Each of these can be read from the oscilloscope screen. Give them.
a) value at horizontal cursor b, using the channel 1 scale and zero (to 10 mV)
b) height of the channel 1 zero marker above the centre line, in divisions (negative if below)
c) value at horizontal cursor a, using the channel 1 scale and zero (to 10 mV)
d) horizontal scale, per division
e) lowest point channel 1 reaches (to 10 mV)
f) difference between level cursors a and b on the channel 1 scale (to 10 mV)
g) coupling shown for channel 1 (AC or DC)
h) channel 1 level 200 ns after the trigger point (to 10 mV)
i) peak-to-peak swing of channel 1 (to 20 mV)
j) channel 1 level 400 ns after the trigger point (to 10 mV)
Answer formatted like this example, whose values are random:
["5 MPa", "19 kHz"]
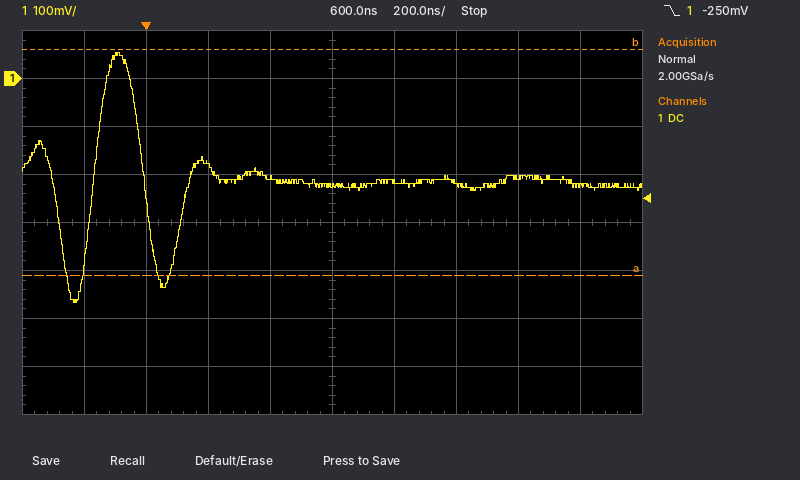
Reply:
["60 mV", "+3.0 div", "-410 mV", "200 ns", "-470 mV", "470 mV", "DC", "-180 mV", "520 mV", "-210 mV"]
